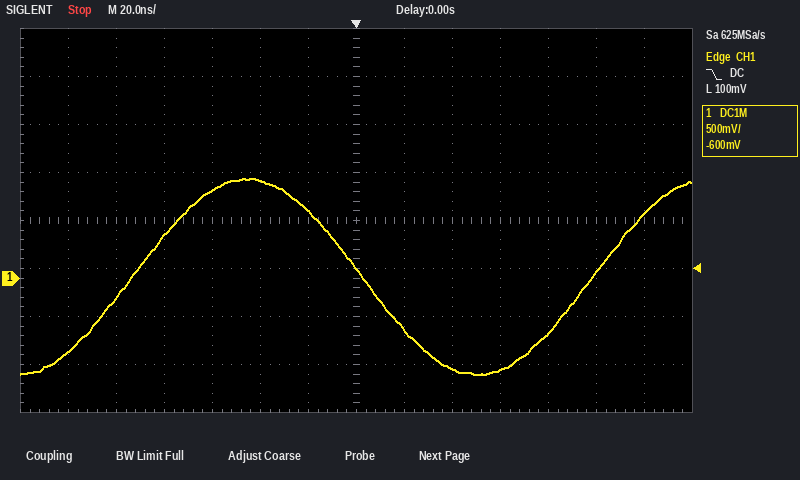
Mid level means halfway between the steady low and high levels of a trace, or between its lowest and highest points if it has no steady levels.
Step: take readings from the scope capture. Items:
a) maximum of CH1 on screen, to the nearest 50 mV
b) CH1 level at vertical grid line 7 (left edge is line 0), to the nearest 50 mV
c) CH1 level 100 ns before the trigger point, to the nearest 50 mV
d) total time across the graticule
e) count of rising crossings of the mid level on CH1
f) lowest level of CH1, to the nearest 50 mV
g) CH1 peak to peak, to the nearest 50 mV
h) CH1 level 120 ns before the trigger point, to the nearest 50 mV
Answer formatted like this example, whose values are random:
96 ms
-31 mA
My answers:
1.05 V
100 mV
-200 mV
280 ns
2
-1.00 V
2.05 V
-750 mV
